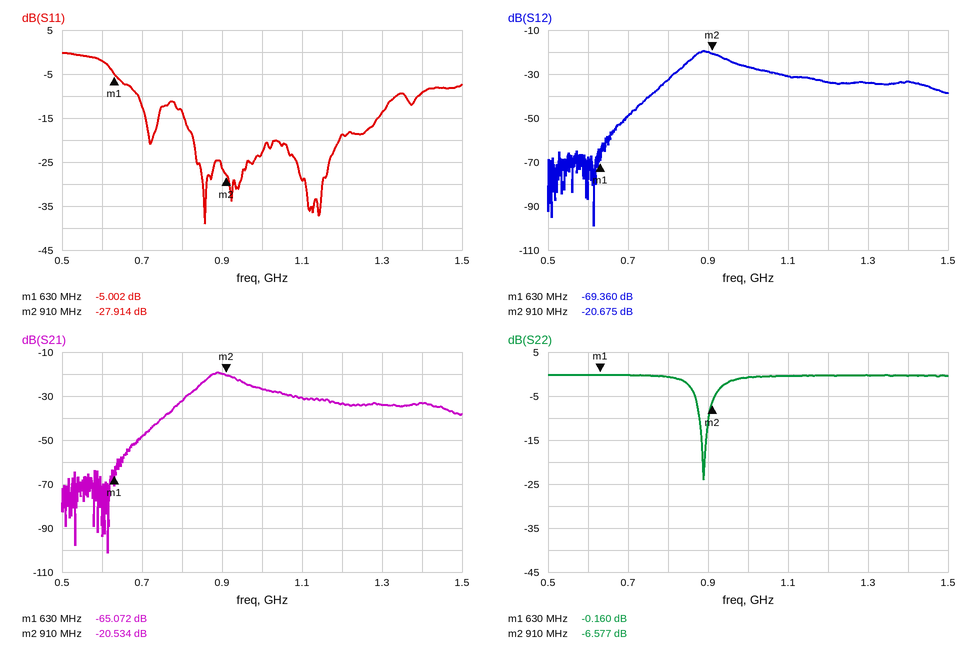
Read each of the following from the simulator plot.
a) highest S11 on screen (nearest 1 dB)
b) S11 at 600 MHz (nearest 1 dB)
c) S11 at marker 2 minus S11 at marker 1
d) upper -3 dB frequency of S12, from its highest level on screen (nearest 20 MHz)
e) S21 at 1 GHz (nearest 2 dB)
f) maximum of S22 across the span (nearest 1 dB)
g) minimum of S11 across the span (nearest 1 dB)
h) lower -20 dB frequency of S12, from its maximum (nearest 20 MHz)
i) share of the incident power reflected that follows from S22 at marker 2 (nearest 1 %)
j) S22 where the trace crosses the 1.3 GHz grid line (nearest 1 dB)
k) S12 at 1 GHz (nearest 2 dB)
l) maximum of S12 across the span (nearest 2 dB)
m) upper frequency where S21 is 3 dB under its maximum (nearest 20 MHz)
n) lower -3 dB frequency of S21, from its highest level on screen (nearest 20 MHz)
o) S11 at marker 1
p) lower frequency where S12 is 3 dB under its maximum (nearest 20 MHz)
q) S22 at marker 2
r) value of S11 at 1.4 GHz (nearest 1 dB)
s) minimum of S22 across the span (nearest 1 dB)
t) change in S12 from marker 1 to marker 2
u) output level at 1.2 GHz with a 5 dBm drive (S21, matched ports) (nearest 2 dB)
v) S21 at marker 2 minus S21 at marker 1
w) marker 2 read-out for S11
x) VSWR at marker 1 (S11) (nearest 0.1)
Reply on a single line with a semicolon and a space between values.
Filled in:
0 dB; -2 dB; -22.912 dB; 940 MHz; -26 dB; 0 dB; -39 dB; 760 MHz; 22 %; 0 dB; -26 dB; -20 dB; 940 MHz; 860 MHz; -5.002 dB; 860 MHz; -6.577 dB; -9 dB; -24 dB; 48.685 dB; -28 dBm; 44.538 dB; -27.914 dB; 3.6
